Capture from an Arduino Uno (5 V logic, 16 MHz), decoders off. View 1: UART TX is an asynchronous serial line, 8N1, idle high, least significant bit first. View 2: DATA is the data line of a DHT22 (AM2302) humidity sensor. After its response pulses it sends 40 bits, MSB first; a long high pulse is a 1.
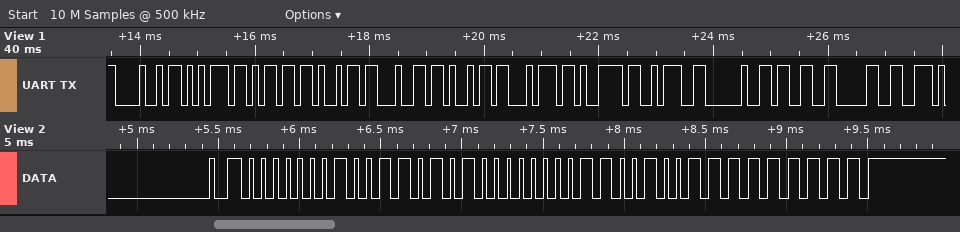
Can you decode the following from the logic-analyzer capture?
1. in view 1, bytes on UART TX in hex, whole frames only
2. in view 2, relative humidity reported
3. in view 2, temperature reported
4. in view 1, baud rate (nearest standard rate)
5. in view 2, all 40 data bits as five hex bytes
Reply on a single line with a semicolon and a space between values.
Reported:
48 75 6D 69 64 69 74 79 3A 20 33 30; 30.9 %; 20.1 °C; 9600 baud; 01 35 00 C9 FF
